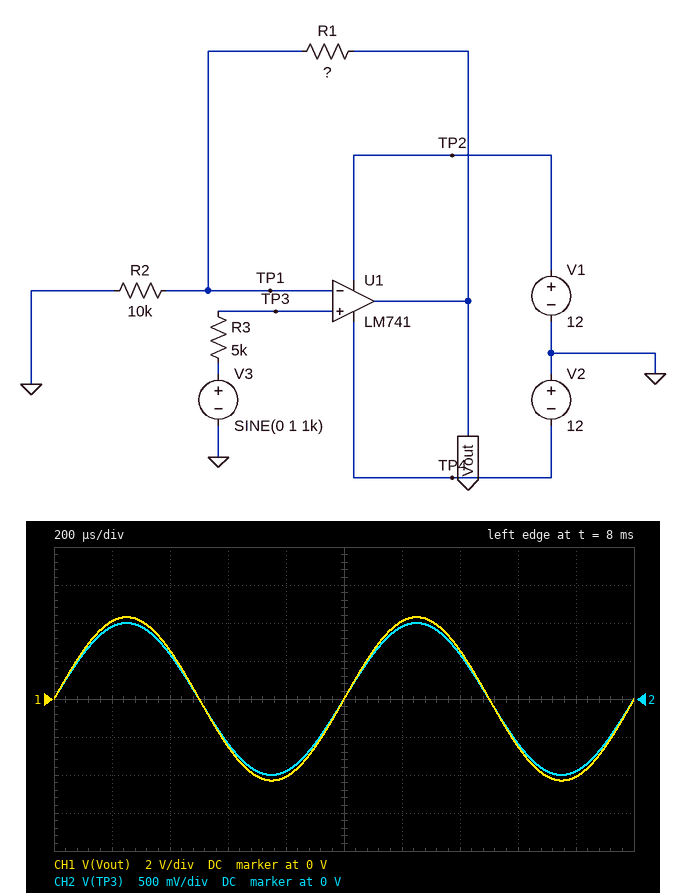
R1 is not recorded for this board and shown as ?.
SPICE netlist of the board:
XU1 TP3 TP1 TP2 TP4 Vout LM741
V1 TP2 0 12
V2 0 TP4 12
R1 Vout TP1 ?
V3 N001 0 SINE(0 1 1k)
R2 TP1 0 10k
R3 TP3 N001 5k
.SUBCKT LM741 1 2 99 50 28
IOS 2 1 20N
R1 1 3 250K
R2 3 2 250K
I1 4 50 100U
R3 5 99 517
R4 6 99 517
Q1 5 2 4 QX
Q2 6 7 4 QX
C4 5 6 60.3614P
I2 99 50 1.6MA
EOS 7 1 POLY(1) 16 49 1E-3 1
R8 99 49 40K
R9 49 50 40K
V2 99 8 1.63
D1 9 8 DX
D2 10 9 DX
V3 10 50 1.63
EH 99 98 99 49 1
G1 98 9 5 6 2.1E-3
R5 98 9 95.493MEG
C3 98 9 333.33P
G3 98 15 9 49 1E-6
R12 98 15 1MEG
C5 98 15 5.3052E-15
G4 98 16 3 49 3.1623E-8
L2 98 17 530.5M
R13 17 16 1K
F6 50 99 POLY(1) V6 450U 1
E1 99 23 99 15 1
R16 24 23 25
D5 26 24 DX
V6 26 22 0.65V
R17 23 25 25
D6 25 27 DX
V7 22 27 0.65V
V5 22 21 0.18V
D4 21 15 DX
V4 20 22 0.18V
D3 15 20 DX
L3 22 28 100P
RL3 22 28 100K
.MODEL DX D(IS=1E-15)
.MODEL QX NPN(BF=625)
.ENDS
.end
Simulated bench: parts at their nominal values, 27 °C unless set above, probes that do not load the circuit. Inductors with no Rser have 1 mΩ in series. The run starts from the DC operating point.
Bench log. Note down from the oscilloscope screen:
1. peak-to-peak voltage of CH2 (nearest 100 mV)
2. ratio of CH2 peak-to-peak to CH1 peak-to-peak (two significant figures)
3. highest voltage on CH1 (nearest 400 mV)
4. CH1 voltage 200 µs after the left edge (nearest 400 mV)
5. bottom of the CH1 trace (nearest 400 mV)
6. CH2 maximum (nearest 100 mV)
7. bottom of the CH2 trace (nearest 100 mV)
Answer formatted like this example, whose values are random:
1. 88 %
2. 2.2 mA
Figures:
1. 2.0 V
2. 0.23
3. 4.4 V
4. 4.0 V
5. -4.4 V
6. 1.0 V
7. -1.0 V
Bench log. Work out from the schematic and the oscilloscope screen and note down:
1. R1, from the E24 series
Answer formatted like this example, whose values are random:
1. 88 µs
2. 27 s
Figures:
1. 33 kΩ
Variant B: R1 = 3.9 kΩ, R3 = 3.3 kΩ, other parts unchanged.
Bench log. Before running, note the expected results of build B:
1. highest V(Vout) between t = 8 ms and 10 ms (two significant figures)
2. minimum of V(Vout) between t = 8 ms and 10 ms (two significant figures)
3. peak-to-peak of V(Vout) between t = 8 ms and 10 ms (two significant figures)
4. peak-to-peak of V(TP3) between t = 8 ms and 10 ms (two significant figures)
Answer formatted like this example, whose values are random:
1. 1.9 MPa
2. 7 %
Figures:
1. 1.4 V
2. -1.4 V
3. 2.8 V
4. 2.0 V
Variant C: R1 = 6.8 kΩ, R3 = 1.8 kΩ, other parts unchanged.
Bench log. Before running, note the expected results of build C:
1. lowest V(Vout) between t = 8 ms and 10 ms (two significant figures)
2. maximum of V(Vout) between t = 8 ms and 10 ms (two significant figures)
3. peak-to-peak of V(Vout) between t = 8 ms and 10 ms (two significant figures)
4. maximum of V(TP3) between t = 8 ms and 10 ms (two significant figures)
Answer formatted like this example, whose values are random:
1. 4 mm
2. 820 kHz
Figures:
1. -1.7 V
2. 1.7 V
3. 3.4 V
4. 1.0 V
